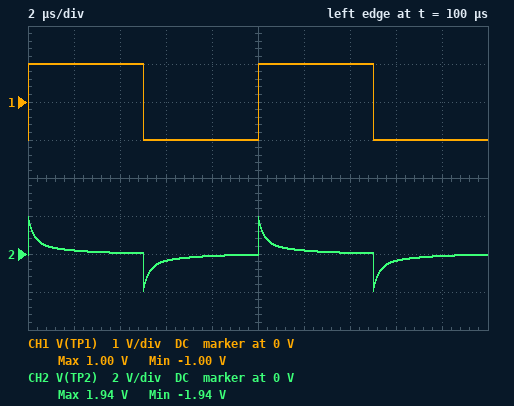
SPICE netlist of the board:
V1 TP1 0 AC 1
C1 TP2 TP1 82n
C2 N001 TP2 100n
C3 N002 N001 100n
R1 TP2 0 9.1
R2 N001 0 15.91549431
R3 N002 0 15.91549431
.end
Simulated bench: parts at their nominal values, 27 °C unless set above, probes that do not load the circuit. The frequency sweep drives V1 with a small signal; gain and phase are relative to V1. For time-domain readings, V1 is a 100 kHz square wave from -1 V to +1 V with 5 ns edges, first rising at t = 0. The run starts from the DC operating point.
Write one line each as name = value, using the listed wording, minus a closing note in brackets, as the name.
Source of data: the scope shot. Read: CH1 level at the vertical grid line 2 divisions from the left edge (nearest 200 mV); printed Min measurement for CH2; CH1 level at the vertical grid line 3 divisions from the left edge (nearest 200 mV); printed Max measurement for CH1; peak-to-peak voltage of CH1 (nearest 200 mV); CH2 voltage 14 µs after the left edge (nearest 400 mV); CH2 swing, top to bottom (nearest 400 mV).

CH1 level at the vertical grid line 2 divisions from the left edge = 1.0 V
printed Min measurement for CH2 = -1.94 V
CH1 level at the vertical grid line 3 divisions from the left edge = -1.0 V
printed Max measurement for CH1 = 1.00 V
peak-to-peak voltage of CH1 = 2.0 V
CH2 voltage 14 µs after the left edge = 0 V
CH2 swing, top to bottom = 4.0 V
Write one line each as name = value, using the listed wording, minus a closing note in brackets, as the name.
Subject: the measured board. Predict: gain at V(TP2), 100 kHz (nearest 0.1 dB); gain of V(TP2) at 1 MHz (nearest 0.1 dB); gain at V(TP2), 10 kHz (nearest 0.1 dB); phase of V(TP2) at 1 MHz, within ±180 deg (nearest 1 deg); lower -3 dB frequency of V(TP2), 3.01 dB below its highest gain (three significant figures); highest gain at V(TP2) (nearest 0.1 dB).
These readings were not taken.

gain at V(TP2), 100 kHz = -9.9 dB
gain of V(TP2) at 1 MHz = -1.2 dB
gain at V(TP2), 10 kHz = -26.7 dB
phase of V(TP2) at 1 MHz, within ±180 deg = 23 deg
lower -3 dB frequency of V(TP2), 3.01 dB below its highest gain = 525 kHz
highest gain at V(TP2) = 0 dB
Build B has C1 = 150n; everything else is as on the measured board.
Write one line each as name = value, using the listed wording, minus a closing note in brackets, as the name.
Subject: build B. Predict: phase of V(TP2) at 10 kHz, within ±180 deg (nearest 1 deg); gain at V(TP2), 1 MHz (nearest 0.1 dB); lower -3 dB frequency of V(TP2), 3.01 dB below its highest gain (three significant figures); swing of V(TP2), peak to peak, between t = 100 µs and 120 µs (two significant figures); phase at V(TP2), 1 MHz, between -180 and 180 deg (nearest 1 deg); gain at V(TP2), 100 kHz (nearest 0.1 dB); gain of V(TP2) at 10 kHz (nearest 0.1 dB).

phase of V(TP2) at 10 kHz, within ±180 deg = 82 deg
gain at V(TP2), 1 MHz = -0.5 dB
lower -3 dB frequency of V(TP2), 3.01 dB below its highest gain = 274 kHz
swing of V(TP2), peak to peak, between t = 100 µs and 120 µs = 3.8 V
phase at V(TP2), 1 MHz, between -180 and 180 deg = 13 deg
gain at V(TP2), 100 kHz = -6.0 dB
gain of V(TP2) at 10 kHz = -21.5 dB
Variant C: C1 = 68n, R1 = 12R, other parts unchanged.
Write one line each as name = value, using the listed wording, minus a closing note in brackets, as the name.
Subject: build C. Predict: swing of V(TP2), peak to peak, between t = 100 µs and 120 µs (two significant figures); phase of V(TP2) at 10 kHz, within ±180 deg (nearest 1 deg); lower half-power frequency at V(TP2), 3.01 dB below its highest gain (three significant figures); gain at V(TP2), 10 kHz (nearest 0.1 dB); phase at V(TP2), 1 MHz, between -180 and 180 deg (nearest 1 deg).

swing of V(TP2), peak to peak, between t = 100 µs and 120 µs = 3.9 V
phase of V(TP2) at 10 kHz, within ±180 deg = 83 deg
lower half-power frequency at V(TP2), 3.01 dB below its highest gain = 572 kHz
gain at V(TP2), 10 kHz = -25.9 dB
phase at V(TP2), 1 MHz, between -180 and 180 deg = 24 deg
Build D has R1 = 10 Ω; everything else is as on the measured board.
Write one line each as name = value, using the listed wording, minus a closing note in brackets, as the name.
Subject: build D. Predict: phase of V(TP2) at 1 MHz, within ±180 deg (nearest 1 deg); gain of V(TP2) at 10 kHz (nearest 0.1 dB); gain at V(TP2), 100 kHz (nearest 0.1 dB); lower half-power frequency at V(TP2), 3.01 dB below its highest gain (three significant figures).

phase of V(TP2) at 1 MHz, within ±180 deg = 22 deg
gain of V(TP2) at 10 kHz = -25.9 dB
gain at V(TP2), 100 kHz = -9.4 dB
lower half-power frequency at V(TP2), 3.01 dB below its highest gain = 507 kHz
